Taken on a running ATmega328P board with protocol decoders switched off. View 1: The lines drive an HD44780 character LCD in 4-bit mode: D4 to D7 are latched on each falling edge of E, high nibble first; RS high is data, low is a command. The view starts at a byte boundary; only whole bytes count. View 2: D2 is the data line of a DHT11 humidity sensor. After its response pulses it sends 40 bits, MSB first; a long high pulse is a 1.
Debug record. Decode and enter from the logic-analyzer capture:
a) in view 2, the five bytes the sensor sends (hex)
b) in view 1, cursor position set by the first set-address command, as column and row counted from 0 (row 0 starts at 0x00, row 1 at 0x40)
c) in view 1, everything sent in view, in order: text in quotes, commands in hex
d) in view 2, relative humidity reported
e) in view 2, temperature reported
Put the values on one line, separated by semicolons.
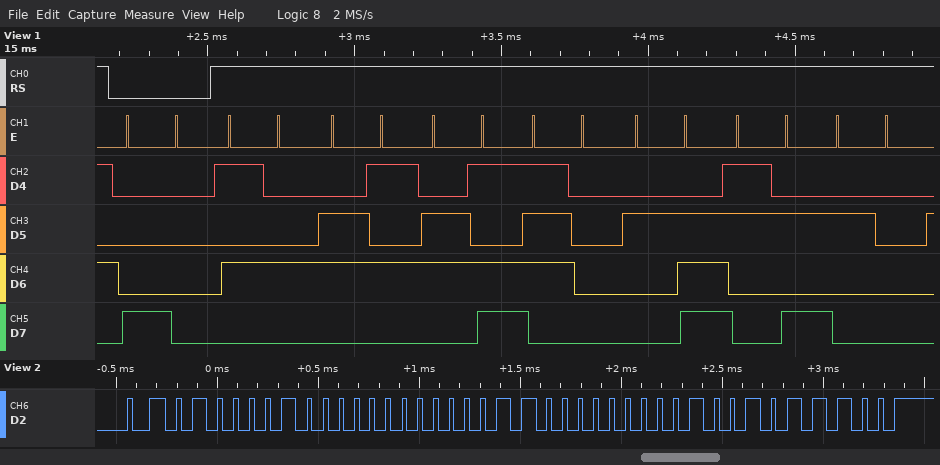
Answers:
42 00 18 02 5C; column 0, row 0; 0x80 "Temp.: "; 66 %; 24.2 °C
